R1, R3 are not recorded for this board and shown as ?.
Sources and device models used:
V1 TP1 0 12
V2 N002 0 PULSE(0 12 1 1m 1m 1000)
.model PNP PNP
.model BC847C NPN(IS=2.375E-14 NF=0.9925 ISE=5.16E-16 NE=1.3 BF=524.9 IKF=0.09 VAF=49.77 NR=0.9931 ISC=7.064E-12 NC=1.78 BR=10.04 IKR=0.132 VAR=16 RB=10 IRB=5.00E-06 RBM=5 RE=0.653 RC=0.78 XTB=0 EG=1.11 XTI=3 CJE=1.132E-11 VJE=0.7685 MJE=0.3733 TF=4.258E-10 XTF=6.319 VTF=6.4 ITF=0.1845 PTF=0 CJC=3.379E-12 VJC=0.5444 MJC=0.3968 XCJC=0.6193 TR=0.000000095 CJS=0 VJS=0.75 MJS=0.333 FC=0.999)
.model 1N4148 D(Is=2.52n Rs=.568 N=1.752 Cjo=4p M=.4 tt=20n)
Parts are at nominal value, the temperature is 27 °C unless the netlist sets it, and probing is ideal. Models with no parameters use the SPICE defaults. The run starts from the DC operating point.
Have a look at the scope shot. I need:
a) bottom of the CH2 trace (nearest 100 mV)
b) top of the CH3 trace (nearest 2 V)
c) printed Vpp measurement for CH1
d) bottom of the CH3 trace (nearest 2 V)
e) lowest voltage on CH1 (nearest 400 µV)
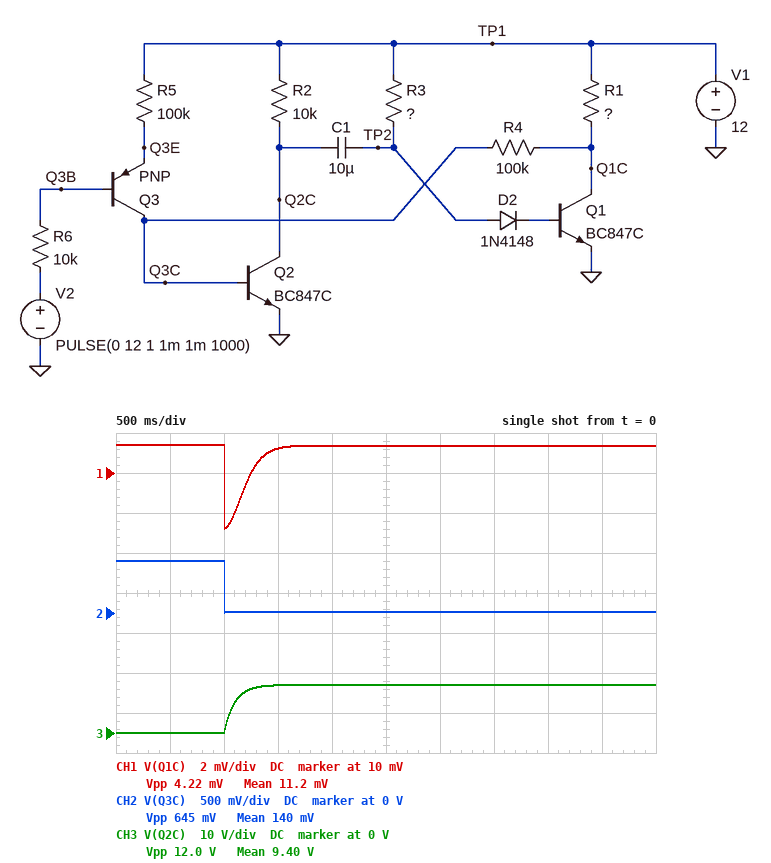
0 V
12 V
4.22 mV
0 V
7.2 mV
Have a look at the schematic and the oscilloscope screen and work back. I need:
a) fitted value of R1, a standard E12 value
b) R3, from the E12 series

12 kΩ
33 kΩ
